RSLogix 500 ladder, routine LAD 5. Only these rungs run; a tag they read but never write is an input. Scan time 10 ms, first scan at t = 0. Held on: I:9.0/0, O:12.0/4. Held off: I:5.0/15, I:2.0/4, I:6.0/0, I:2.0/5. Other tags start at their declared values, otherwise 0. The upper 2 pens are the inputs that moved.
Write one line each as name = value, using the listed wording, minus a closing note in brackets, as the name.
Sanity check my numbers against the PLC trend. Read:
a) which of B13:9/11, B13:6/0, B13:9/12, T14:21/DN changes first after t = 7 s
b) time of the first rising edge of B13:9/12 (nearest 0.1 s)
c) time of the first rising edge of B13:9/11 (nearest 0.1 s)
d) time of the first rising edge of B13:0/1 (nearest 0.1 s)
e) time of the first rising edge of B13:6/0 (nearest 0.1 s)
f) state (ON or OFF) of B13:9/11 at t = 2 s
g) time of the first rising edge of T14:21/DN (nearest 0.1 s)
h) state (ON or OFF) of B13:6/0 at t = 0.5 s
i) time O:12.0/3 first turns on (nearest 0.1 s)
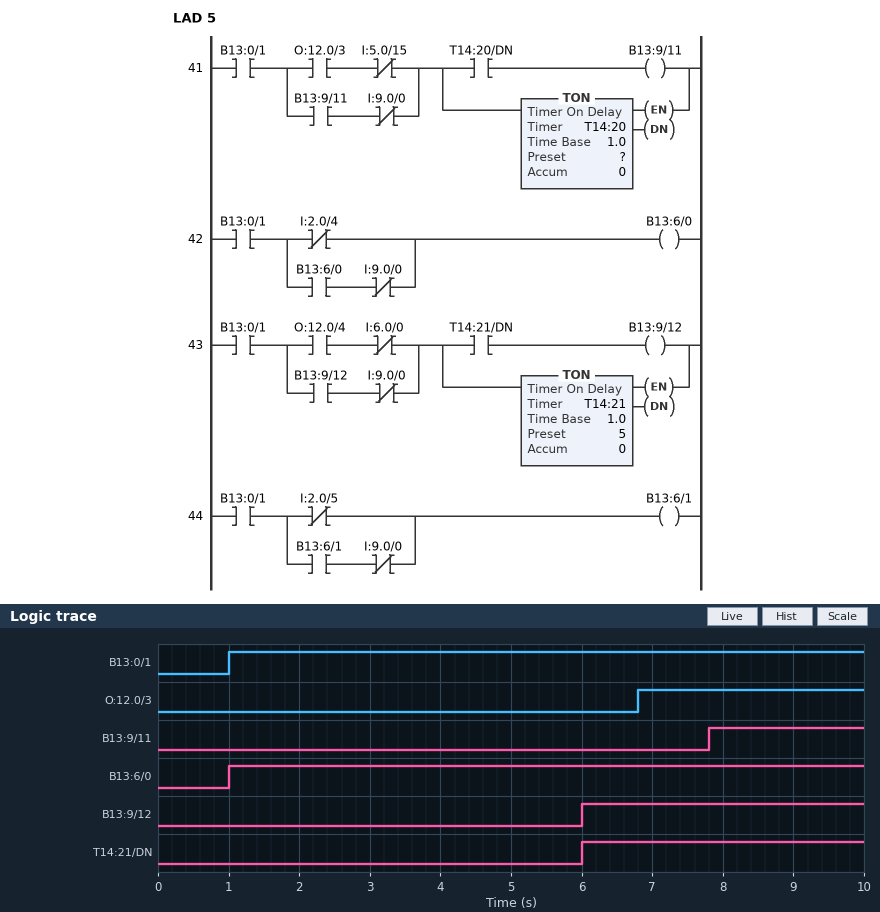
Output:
which of B13:9/11, B13:6/0, B13:9/12, T14:21/DN changes first after t = 7 s = B13:9/11
time of the first rising edge of B13:9/12 = 6.0 s
time of the first rising edge of B13:9/11 = 7.8 s
time of the first rising edge of B13:0/1 = 1.0 s
time of the first rising edge of B13:6/0 = 1.0 s
state (ON or OFF) of B13:9/11 at t = 2 s = OFF
time of the first rising edge of T14:21/DN = 6.0 s
state (ON or OFF) of B13:6/0 at t = 0.5 s = OFF
time O:12.0/3 first turns on = 6.8 s
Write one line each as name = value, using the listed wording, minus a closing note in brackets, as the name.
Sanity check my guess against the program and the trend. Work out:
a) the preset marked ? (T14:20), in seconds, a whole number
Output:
the preset marked ? (T14:20), in seconds, a whole number = 1 s
